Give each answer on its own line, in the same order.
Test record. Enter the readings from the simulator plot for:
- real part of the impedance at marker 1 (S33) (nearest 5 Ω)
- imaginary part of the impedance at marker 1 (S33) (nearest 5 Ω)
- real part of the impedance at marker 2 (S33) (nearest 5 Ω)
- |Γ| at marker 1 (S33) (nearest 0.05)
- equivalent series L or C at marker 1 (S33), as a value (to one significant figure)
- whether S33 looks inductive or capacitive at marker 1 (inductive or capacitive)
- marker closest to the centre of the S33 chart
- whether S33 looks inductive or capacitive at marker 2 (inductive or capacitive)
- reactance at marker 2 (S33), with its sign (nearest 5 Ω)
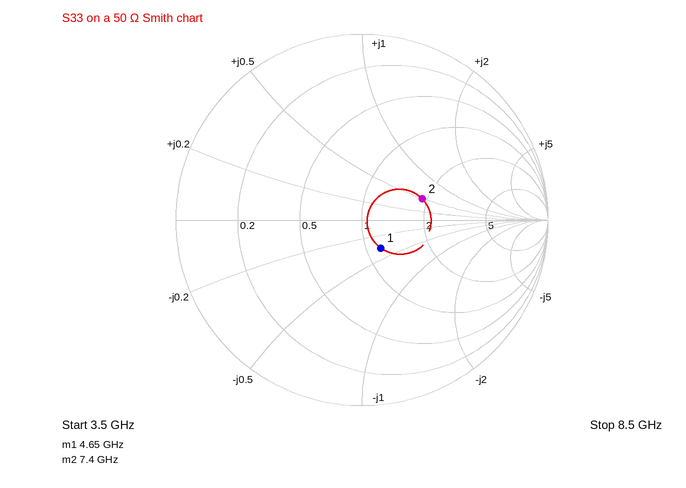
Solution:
60 Ω
-20 Ω
95 Ω
0.20
2 pF
capacitive
marker 1
inductive
+25 Ω
